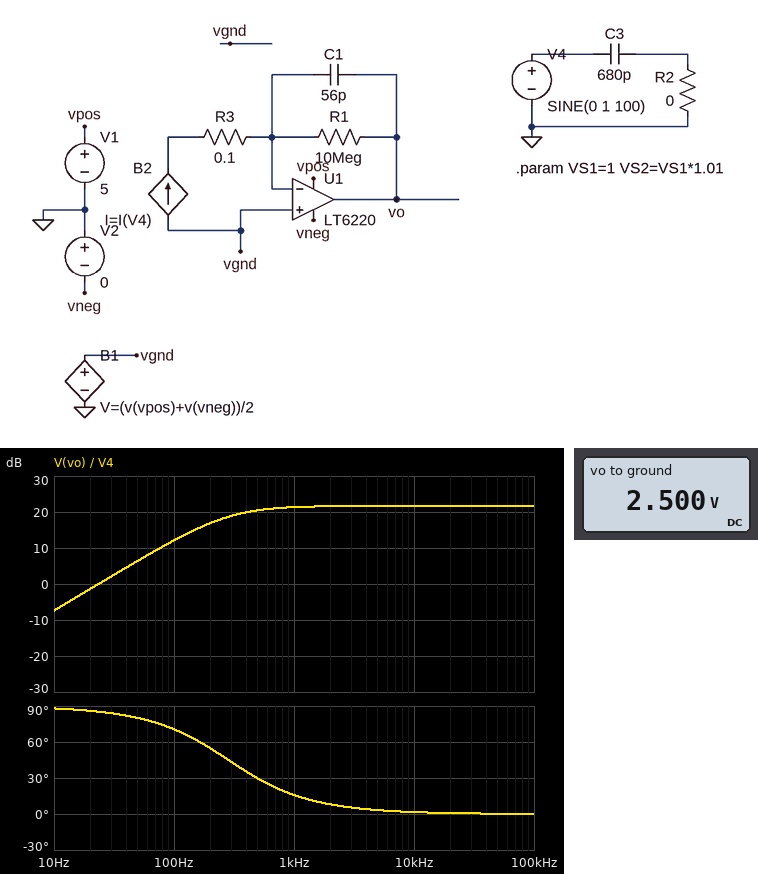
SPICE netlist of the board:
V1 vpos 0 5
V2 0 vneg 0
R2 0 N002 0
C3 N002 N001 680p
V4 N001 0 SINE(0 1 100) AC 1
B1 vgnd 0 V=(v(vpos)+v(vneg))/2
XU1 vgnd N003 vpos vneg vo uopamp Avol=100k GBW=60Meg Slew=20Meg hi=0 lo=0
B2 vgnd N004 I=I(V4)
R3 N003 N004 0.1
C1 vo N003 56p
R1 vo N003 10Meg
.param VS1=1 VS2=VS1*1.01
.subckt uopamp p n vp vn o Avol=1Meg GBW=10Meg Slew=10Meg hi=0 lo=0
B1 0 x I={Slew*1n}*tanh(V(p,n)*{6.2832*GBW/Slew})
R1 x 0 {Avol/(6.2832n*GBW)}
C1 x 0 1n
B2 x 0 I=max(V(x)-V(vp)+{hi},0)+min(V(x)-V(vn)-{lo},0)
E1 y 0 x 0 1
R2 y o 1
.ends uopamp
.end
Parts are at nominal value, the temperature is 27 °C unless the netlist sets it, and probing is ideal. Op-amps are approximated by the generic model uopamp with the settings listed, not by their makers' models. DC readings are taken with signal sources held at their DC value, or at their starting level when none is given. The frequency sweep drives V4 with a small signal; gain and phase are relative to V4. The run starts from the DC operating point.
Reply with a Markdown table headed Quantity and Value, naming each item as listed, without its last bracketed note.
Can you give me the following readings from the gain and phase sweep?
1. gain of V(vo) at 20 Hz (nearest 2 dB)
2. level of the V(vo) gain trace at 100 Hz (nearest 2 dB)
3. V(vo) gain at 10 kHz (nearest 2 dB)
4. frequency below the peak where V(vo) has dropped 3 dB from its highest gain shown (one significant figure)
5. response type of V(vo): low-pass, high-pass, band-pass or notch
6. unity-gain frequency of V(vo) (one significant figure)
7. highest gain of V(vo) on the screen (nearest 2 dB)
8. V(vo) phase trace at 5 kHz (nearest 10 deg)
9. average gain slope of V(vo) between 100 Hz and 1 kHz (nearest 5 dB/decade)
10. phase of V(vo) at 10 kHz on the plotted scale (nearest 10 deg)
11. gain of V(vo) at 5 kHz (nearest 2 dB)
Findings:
| Quantity | Value |
|---|---|
| gain of V(vo) at 20 Hz | -2 dB |
| level of the V(vo) gain trace at 100 Hz | 12 dB |
| V(vo) gain at 10 kHz | 22 dB |
| frequency below the peak where V(vo) has dropped 3 dB from its highest gain shown | 300 Hz |
| response type of V(vo): low-pass, high-pass, band-pass or notch | high-pass |
| unity-gain frequency of V(vo) | 20 Hz |
| highest gain of V(vo) on the screen | 22 dB |
| V(vo) phase trace at 5 kHz | 0 deg |
| average gain slope of V(vo) between 100 Hz and 1 kHz | 10 dB/decade |
| phase of V(vo) at 10 kHz on the plotted scale | 0 deg |
| gain of V(vo) at 5 kHz | 22 dB |
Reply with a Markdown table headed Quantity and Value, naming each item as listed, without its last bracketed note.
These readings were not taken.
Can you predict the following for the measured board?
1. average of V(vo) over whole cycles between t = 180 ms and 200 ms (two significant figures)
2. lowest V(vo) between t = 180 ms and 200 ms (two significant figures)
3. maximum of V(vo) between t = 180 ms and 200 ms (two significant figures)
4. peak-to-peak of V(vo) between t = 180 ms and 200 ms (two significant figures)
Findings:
| Quantity | Value |
|---|---|
| average of V(vo) over whole cycles between t = 180 ms and 200 ms | 2.5 V |
| lowest V(vo) between t = 180 ms and 200 ms | -20 mV |
| maximum of V(vo) between t = 180 ms and 200 ms | 5.0 V |
| peak-to-peak of V(vo) between t = 180 ms and 200 ms | 5.0 V |
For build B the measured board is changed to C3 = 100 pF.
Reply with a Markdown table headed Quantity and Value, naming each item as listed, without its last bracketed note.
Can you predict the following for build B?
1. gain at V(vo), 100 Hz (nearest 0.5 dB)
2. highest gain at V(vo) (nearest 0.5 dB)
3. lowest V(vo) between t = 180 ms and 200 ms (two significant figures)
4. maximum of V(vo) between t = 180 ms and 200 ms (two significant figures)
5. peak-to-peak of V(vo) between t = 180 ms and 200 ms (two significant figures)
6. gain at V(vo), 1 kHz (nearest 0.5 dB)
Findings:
| Quantity | Value |
|---|---|
| gain at V(vo), 100 Hz | -4.5 dB |
| highest gain at V(vo) | 5.0 dB |
| lowest V(vo) between t = 180 ms and 200 ms | 1.9 V |
| maximum of V(vo) between t = 180 ms and 200 ms | 3.1 V |
| peak-to-peak of V(vo) between t = 180 ms and 200 ms | 1.2 V |
| gain at V(vo), 1 kHz | 4.5 dB |
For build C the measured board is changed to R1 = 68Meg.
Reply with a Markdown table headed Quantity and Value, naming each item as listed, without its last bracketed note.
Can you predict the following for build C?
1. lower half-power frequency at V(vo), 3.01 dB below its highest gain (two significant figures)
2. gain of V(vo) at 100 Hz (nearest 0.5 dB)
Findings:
| Quantity | Value |
|---|---|
| lower half-power frequency at V(vo), 3.01 dB below its highest gain | 42 Hz |
| gain of V(vo) at 100 Hz | 21.0 dB |
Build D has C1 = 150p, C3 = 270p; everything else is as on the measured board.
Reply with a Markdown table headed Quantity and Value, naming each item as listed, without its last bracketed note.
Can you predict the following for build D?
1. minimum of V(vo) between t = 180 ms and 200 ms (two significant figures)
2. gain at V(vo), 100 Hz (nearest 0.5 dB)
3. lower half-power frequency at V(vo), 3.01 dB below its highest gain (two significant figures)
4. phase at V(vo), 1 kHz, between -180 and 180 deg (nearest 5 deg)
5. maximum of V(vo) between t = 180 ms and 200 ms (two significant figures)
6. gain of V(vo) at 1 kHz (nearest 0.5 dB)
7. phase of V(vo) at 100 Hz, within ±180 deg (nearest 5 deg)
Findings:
| Quantity | Value |
|---|---|
| minimum of V(vo) between t = 180 ms and 200 ms | 1.3 V |
| gain at V(vo), 100 Hz | 2.0 dB |
| lower half-power frequency at V(vo), 3.01 dB below its highest gain | 110 Hz |
| phase at V(vo), 1 kHz, between -180 and 180 deg | 5 deg |
| maximum of V(vo) between t = 180 ms and 200 ms | 3.7 V |
| gain of V(vo) at 1 kHz | 5.0 dB |
| phase of V(vo) at 100 Hz, within ±180 deg | 45 deg |
